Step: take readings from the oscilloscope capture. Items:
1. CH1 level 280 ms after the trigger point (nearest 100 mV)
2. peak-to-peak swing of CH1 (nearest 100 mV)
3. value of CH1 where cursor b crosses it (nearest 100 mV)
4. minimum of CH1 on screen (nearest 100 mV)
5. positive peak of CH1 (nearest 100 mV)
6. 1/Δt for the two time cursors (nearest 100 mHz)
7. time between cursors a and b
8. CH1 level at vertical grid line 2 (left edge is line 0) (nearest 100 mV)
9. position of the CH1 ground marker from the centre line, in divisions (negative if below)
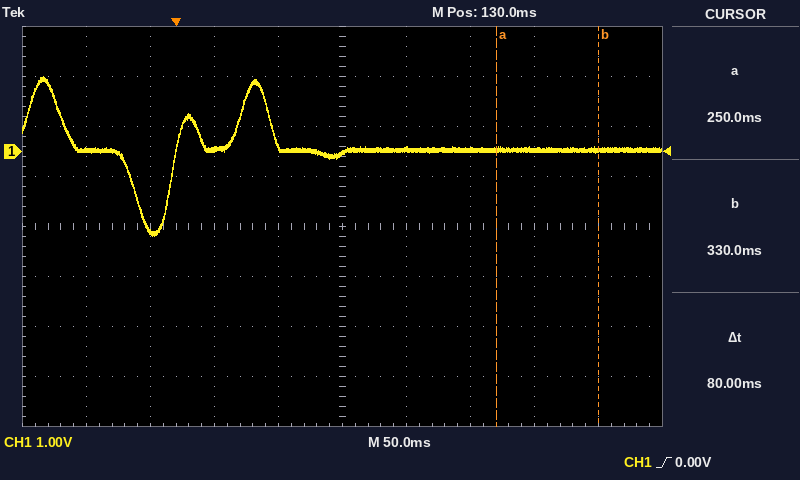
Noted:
0.0 V
3.2 V
0.0 V
-1.7 V
1.5 V
12.5 Hz
80 ms
-1.6 V
+1.5 div
